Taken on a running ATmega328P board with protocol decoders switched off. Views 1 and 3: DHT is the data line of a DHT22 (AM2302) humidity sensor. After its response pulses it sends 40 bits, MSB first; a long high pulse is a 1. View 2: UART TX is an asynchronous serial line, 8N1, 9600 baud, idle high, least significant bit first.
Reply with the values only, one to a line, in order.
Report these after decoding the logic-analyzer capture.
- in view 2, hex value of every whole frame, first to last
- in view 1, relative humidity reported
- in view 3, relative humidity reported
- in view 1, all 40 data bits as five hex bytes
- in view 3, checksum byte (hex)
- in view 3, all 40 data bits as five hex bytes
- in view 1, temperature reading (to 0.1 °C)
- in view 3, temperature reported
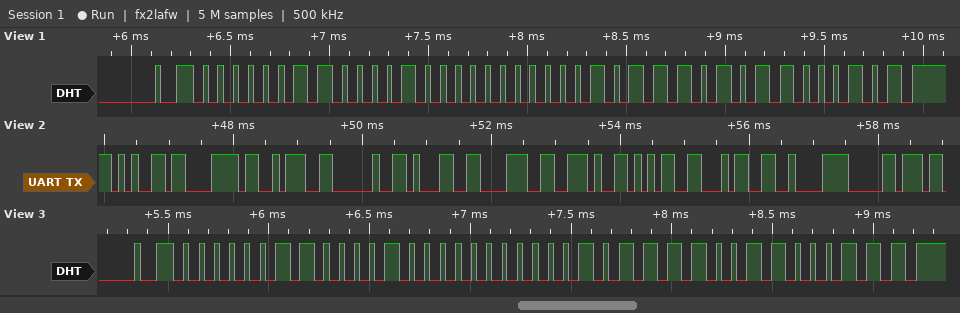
65 78 3A 20 31 38 2E 35 34 C2 B0
77.6 %
77.6 %
03 08 00 BA C5
0xC7
03 08 00 BC C7
18.6 °C
18.8 °C
